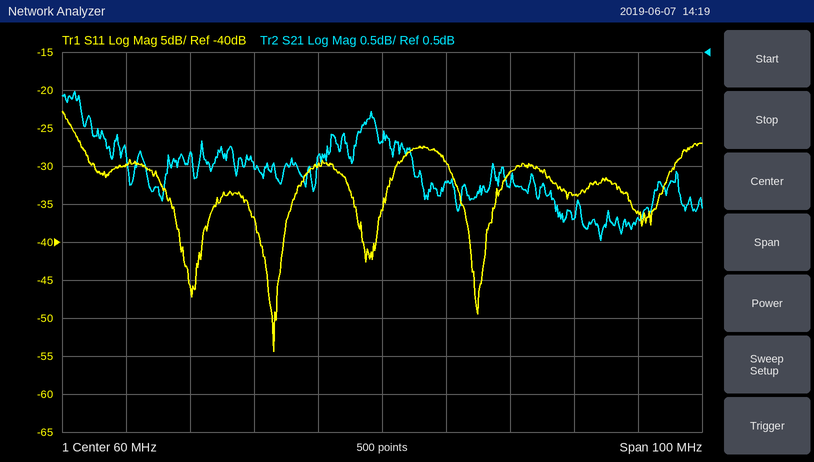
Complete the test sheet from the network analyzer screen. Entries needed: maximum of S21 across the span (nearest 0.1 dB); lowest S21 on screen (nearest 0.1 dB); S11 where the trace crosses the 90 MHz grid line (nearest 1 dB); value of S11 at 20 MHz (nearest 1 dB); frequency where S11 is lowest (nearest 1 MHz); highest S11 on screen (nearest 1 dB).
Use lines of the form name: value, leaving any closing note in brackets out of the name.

maximum of S21 across the span: 0.0 dB
lowest S21 on screen: -2.0 dB
S11 where the trace crosses the 90 MHz grid line: -34 dB
value of S11 at 20 MHz: -30 dB
frequency where S11 is lowest: 43 MHz
highest S11 on screen: -23 dB
